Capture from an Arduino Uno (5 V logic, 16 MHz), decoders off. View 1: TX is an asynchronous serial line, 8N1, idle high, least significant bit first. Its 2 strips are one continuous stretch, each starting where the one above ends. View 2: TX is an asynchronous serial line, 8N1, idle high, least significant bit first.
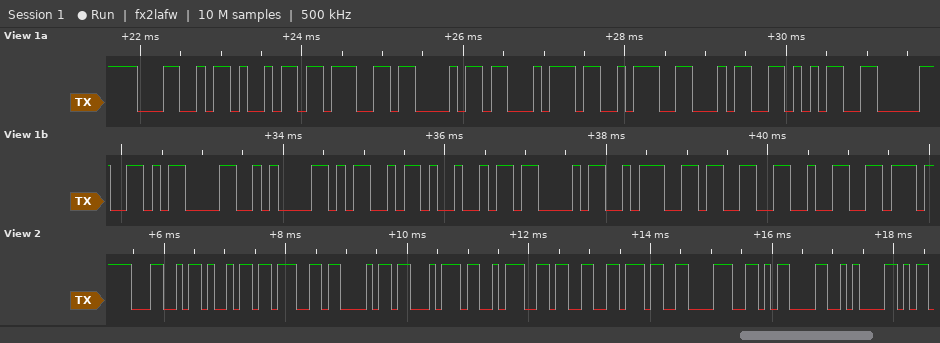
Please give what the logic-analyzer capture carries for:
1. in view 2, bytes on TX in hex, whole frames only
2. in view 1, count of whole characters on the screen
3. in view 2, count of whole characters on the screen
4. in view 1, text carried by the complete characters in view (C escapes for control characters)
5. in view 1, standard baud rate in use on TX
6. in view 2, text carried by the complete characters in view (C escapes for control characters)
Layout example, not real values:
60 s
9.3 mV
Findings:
4C 69 67 68 74 3A 33 37 38 0D 0A
17
11
"Light:450\r\nMIC:32"
9600 baud
"Light:378\r\n"
